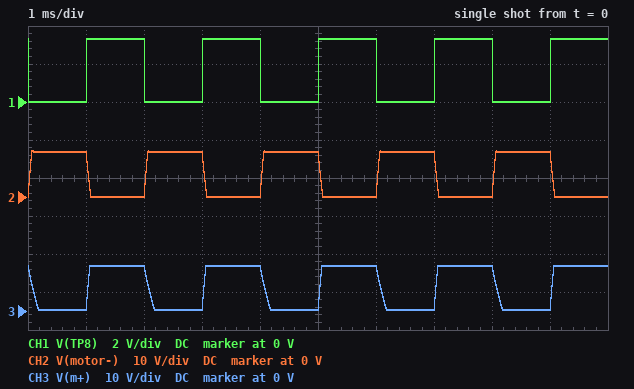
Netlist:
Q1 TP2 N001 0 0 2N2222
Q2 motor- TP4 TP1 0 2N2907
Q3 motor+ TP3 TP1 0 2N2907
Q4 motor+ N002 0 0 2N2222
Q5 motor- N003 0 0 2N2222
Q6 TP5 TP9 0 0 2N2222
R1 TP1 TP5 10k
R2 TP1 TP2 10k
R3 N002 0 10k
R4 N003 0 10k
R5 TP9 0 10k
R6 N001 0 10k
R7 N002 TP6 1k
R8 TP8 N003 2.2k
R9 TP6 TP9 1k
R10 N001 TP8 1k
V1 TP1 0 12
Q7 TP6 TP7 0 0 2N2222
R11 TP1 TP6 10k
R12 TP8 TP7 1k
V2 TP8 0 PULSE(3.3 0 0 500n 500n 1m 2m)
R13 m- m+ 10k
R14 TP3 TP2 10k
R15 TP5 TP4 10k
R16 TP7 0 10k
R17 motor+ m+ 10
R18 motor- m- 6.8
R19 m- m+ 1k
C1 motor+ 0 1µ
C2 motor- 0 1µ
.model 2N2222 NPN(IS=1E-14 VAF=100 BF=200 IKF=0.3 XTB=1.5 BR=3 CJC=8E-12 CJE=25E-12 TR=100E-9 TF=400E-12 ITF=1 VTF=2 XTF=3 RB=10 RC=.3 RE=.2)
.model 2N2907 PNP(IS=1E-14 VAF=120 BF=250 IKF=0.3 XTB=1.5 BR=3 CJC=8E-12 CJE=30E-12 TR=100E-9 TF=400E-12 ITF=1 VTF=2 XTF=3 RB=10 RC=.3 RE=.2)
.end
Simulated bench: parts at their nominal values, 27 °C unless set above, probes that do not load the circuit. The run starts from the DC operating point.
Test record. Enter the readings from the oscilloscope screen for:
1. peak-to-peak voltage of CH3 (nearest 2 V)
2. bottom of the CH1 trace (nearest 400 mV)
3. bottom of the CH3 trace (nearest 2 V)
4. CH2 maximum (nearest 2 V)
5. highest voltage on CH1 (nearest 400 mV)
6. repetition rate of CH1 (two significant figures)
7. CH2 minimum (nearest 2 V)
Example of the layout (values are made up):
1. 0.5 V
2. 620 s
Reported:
1. 12 V
2. 0 V
3. 0 V
4. 12 V
5. 3.2 V
6. 500 Hz
7. 0 V
